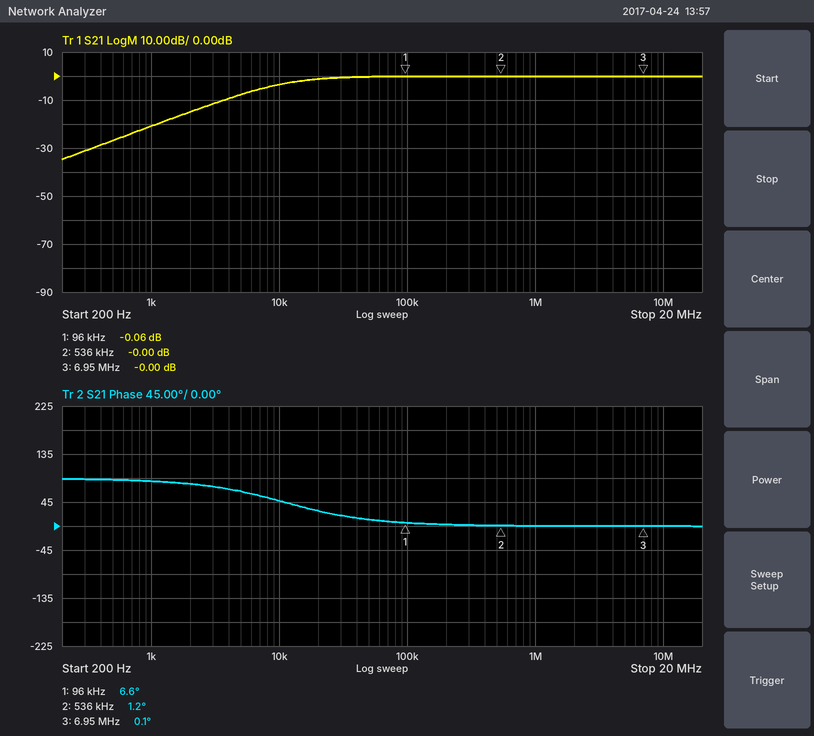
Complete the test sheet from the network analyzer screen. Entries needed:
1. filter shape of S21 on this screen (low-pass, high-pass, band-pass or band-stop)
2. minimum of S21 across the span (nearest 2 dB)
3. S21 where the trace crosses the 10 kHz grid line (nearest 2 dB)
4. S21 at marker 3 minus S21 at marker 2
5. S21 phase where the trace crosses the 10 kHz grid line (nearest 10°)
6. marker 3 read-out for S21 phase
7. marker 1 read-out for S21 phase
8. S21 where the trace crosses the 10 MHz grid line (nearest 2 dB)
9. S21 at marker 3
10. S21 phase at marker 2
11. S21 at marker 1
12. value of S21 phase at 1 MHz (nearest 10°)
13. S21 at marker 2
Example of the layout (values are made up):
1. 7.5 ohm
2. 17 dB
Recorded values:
1. high-pass
2. -34 dB
3. -4 dB
4. 0.00 dB
5. 50°
6. 0.1°
7. 6.6°
8. 0 dB
9. -0.00 dB
10. 1.2°
11. -0.06 dB
12. 0°
13. -0.00 dB
